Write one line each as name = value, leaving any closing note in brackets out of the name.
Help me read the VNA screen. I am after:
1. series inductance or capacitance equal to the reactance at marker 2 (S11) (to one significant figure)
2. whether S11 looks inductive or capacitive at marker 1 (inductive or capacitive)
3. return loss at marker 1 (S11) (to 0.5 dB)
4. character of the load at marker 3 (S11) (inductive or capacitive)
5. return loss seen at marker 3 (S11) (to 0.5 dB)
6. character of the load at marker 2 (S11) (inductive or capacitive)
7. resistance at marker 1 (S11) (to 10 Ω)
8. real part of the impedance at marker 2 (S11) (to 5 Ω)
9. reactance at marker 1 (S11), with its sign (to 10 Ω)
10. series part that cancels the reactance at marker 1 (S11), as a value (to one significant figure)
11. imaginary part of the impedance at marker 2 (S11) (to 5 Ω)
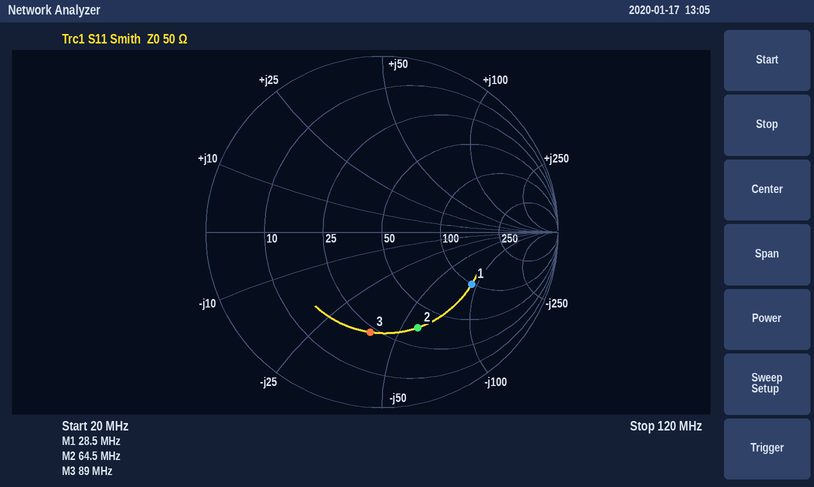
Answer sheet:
series inductance or capacitance equal to the reactance at marker 2 (S11) = 40 pF
whether S11 looks inductive or capacitive at marker 1 = capacitive
return loss at marker 1 (S11) = 4.5 dB
character of the load at marker 3 (S11) = capacitive
return loss seen at marker 3 (S11) = 5.0 dB
character of the load at marker 2 (S11) = capacitive
resistance at marker 1 (S11) = 100 Ω
real part of the impedance at marker 2 (S11) = 35 Ω
reactance at marker 1 (S11), with its sign = -90 Ω
series part that cancels the reactance at marker 1 (S11), as a value = 500 nH
imaginary part of the impedance at marker 2 (S11) = -60 Ω
